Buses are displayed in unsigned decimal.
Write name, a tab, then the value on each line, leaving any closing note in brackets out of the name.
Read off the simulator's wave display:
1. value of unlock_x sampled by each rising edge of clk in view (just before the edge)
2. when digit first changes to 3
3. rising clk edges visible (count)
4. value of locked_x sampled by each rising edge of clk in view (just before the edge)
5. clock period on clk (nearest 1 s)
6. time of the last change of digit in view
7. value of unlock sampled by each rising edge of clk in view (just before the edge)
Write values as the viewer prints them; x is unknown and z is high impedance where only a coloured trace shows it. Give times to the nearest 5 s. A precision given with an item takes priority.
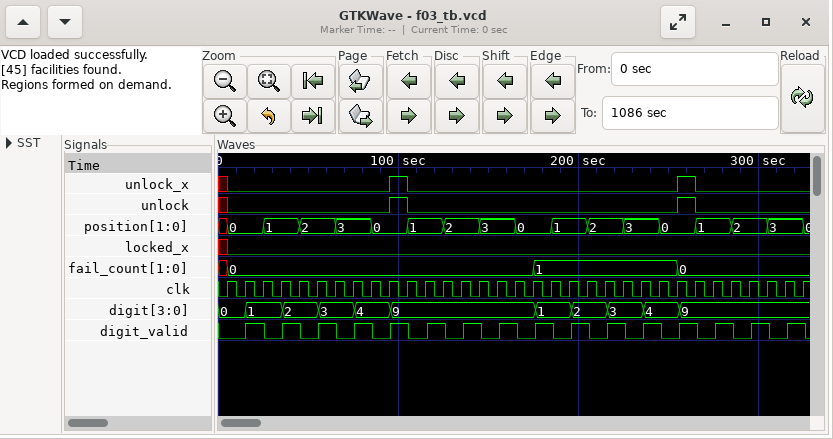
value of unlock_x sampled by each rising edge of clk in view	x 0 0 0 0 0 0 0 0 0 1 0 0 0 0 0 0 0 0 0 0 0 0 0 0 0 1 0 0 0 0 0 0
when digit first changes to 3	55 s
rising clk edges visible	33
value of locked_x sampled by each rising edge of clk in view	x 0 0 0 0 0 0 0 0 0 0 0 0 0 0 0 0 0 0 0 0 0 0 0 0 0 0 0 0 0 0 0 0
clock period on clk	10 s
time of the last change of digit in view	255 s
value of unlock sampled by each rising edge of clk in view	x 0 0 0 0 0 0 0 0 0 1 0 0 0 0 0 0 0 0 0 0 0 0 0 0 0 1 0 0 0 0 0 0
